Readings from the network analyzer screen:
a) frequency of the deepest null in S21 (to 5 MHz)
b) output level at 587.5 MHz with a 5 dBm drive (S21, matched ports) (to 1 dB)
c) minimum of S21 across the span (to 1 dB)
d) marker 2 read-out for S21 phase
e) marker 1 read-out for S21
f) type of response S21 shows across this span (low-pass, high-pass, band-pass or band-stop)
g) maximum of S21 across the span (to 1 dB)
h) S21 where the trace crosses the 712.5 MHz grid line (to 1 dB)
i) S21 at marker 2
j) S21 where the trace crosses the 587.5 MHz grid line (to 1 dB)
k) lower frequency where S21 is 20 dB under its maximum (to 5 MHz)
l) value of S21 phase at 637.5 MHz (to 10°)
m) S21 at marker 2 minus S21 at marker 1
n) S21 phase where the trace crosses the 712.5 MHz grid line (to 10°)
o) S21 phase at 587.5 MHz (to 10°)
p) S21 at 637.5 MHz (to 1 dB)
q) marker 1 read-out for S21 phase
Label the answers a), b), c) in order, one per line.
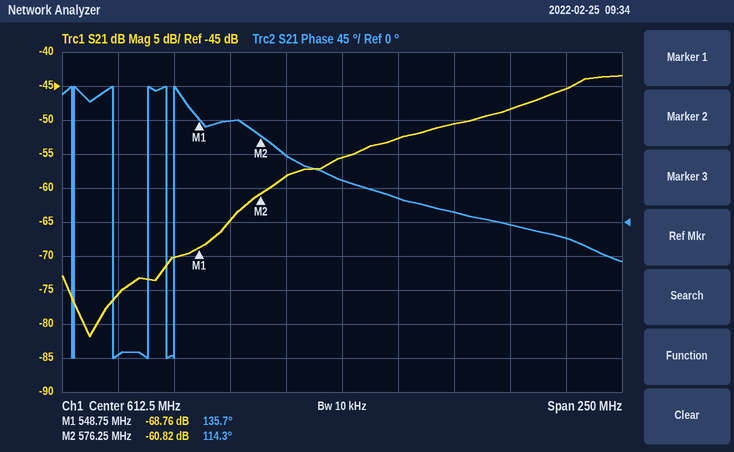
a) 500 MHz
b) -53 dBm
c) -82 dB
d) 114.3°
e) -68.76 dB
f) high-pass
g) -43 dB
h) -45 dB
i) -60.82 dB
j) -58 dB
k) 565 MHz
l) 30°
m) 7.94 dB
n) -20°
o) 90°
p) -53 dB
q) 135.7°
